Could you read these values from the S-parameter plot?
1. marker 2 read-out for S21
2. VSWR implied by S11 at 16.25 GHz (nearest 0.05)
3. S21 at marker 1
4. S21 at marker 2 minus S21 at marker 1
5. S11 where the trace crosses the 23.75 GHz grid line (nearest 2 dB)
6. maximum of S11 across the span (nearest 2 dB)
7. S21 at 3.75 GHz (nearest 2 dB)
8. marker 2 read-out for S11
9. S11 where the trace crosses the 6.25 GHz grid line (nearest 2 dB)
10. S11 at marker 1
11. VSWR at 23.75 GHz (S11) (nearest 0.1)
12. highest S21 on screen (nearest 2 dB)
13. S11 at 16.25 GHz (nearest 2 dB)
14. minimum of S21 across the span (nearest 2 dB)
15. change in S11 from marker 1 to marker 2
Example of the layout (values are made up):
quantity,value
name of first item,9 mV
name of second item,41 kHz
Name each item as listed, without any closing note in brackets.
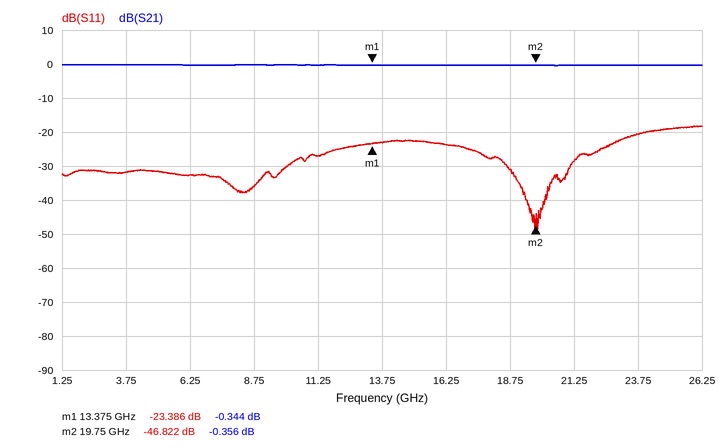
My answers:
quantity,value
marker 2 read-out for S21,-0.356 dB
VSWR implied by S11 at 16.25 GHz,1.15
S21 at marker 1,-0.344 dB
S21 at marker 2 minus S21 at marker 1,-0.012 dB
S11 where the trace crosses the 23.75 GHz grid line,-20 dB
maximum of S11 across the span,-18 dB
S21 at 3.75 GHz,0 dB
marker 2 read-out for S11,-46.822 dB
S11 where the trace crosses the 6.25 GHz grid line,-32 dB
S11 at marker 1,-23.386 dB
VSWR at 23.75 GHz (S11),1.2
highest S21 on screen,0 dB
S11 at 16.25 GHz,-24 dB
minimum of S21 across the span,0 dB
change in S11 from marker 1 to marker 2,-23.436 dB
